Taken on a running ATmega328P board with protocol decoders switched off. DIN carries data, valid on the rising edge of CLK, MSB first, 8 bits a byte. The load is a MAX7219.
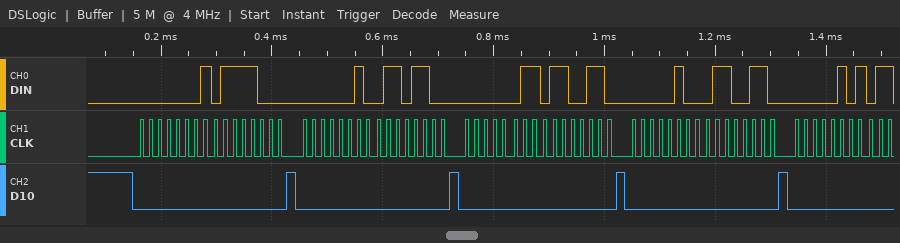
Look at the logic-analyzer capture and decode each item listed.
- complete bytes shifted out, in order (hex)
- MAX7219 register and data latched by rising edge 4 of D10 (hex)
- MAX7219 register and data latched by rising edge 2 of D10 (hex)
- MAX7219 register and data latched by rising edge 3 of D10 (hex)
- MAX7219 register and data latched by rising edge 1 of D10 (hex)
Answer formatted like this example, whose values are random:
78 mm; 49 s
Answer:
01 78 02 6C 03 66 04 66 05; register 0x4, data 0x66; register 0x2, data 0x6C; register 0x3, data 0x66; register 0x1, data 0x78
